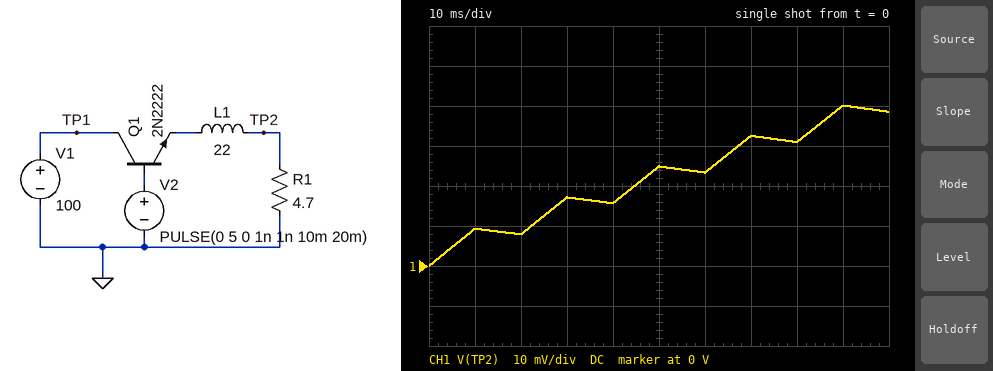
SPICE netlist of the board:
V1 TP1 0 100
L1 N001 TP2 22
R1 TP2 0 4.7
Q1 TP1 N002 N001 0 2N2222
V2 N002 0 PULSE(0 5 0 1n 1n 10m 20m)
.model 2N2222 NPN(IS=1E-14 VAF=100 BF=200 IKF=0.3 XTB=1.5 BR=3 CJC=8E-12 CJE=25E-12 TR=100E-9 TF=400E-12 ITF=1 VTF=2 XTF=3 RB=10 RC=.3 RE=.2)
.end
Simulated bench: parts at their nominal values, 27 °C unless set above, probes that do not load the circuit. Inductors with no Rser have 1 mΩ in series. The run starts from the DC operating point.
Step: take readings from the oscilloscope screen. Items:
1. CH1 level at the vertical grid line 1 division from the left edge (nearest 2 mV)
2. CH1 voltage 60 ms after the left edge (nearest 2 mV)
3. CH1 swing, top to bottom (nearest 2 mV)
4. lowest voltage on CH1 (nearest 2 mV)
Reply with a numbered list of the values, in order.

1. 10 mV
2. 24 mV
3. 40 mV
4. 0 V
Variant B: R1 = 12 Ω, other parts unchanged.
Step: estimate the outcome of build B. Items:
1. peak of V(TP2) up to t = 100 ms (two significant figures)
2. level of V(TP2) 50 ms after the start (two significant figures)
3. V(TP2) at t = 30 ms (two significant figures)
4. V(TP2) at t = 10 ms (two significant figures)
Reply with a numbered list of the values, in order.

1. 100 mV
2. 63 mV
3. 44 mV
4. 24 mV
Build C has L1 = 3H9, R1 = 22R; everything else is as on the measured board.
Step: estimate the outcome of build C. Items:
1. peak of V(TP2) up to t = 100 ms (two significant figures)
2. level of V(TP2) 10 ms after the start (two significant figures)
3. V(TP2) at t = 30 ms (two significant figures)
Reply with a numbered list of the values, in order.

1. 820 mV
2. 240 mV
3. 410 mV
